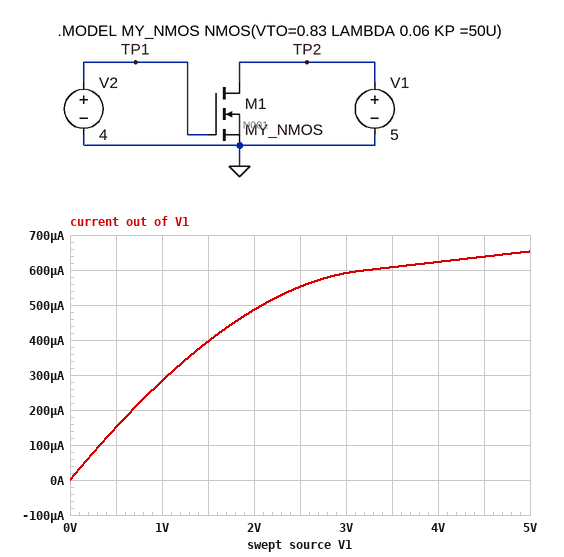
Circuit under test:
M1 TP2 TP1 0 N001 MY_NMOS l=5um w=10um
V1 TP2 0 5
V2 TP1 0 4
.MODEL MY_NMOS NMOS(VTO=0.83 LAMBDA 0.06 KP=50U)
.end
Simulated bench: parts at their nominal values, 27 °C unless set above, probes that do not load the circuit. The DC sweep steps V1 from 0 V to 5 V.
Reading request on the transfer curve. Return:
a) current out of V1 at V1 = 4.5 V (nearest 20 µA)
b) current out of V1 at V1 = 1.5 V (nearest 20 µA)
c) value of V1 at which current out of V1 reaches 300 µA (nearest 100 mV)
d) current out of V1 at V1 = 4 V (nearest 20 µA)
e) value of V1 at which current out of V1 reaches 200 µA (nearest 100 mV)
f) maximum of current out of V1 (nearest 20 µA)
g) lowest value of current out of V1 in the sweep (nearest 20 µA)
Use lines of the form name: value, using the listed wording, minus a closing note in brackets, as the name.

current out of V1 at V1 = 4.5 V: 640 µA
current out of V1 at V1 = 1.5 V: 400 µA
value of V1 at which current out of V1 reaches 300 µA: 1.1 V
current out of V1 at V1 = 4 V: 620 µA
value of V1 at which current out of V1 reaches 200 µA: 700 mV
maximum of current out of V1: 660 µA
lowest value of current out of V1 in the sweep: 0 A
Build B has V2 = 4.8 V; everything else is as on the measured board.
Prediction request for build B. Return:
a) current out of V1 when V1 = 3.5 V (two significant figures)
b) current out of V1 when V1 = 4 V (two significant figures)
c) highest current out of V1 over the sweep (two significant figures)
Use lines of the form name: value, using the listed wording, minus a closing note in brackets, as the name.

current out of V1 when V1 = 3.5 V: 940 µA
current out of V1 when V1 = 4 V: 980 µA
highest current out of V1 over the sweep: 1.0 mA
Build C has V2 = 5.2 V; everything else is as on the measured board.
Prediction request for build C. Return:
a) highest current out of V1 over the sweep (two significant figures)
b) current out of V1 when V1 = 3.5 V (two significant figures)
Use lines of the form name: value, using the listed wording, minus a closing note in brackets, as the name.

highest current out of V1 over the sweep: 1.2 mA
current out of V1 when V1 = 3.5 V: 1.1 mA
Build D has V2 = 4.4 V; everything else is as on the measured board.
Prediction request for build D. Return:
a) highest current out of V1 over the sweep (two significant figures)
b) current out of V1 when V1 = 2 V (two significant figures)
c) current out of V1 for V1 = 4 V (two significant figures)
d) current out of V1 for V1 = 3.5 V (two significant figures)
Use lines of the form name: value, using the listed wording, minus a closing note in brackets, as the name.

highest current out of V1 over the sweep: 830 µA
current out of V1 when V1 = 2 V: 580 µA
current out of V1 for V1 = 4 V: 790 µA
current out of V1 for V1 = 3.5 V: 770 µA
